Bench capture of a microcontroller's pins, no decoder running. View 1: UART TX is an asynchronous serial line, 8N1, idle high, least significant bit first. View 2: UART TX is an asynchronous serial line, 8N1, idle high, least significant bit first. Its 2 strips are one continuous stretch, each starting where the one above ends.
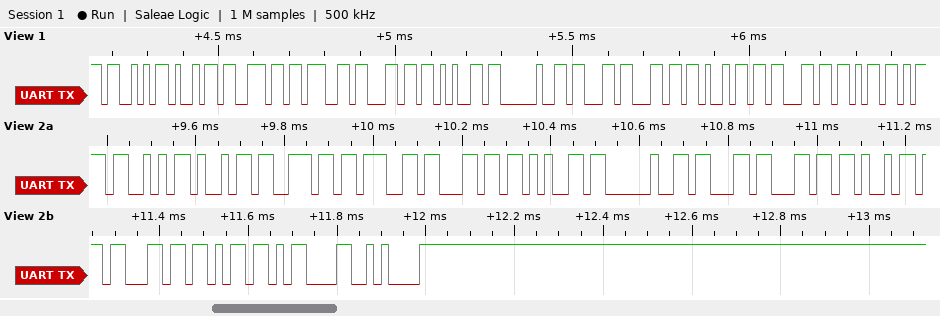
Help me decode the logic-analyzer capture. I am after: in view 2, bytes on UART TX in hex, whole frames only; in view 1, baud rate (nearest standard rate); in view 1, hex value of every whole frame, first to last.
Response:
53 69 6E 67 6C 65 20 63 6C 69 63 6B 0D 0A
57600 baud
53 69 6E 67 6C 65 20 63 6C 69 63 6B
